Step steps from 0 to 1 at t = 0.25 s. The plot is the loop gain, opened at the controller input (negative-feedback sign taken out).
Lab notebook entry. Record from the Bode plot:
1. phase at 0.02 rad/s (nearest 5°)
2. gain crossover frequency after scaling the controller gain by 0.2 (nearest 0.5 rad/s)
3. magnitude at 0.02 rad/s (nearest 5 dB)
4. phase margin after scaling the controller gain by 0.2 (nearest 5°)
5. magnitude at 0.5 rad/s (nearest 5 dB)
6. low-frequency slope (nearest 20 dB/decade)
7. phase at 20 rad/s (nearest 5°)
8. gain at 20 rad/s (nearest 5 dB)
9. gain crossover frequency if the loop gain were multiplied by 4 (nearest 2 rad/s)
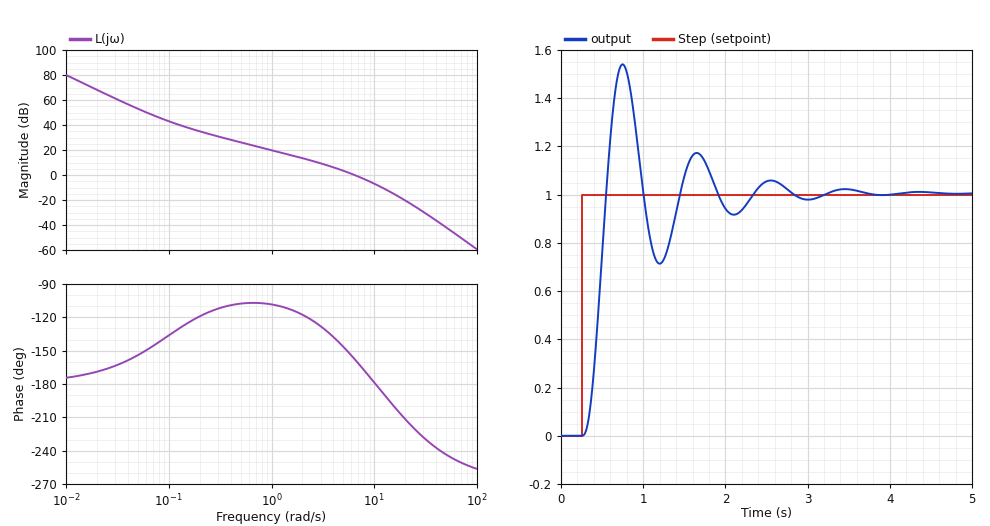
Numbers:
-170°
2.0 rad/s
70 dB
65°
25 dB
-40 dB/decade
-210°
-20 dB
14 rad/s
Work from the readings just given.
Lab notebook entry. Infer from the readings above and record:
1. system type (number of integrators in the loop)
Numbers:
2
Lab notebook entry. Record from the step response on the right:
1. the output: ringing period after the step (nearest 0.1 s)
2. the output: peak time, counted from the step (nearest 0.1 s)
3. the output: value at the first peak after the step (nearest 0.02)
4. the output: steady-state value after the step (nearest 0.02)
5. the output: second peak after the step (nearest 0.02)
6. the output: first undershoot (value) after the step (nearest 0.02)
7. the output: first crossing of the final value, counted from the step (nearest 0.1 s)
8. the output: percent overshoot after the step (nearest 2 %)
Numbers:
0.9 s
0.5 s
1.54
1.00
1.18
0.72
0.3 s
54 %
